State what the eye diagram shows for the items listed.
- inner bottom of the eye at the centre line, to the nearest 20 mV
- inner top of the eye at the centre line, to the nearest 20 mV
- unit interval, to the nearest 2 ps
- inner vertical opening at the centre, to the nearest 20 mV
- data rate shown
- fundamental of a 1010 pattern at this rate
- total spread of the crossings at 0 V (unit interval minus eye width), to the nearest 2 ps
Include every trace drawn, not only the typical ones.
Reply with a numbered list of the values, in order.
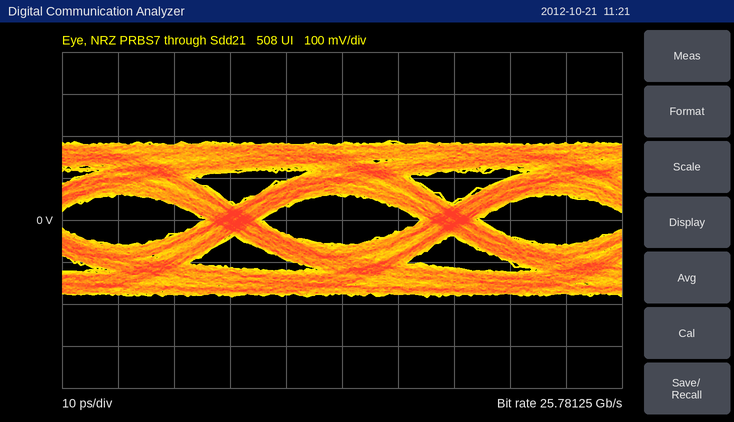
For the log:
1. -60 mV
2. 60 mV
3. 38 ps
4. 120 mV
5. 25.78125 Gb/s
6. 12.89062 GHz
7. 10 ps
